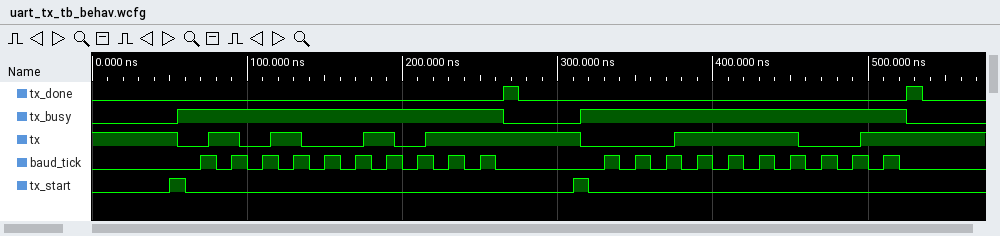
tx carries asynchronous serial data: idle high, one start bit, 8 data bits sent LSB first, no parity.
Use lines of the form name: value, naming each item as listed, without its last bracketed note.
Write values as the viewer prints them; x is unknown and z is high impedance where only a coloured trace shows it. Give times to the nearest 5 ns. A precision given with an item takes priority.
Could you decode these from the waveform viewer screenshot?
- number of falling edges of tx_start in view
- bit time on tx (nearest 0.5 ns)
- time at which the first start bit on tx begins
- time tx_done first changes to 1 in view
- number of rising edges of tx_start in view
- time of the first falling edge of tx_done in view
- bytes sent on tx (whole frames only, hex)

number of falling edges of tx_start in view: 2
bit time on tx: 20 ns
time at which the first start bit on tx begins: 55 ns
time tx_done first changes to 1 in view: 265 ns
number of rising edges of tx_start in view: 2
time of the first falling edge of tx_done in view: 275 ns
bytes sent on tx: A5, 3C
